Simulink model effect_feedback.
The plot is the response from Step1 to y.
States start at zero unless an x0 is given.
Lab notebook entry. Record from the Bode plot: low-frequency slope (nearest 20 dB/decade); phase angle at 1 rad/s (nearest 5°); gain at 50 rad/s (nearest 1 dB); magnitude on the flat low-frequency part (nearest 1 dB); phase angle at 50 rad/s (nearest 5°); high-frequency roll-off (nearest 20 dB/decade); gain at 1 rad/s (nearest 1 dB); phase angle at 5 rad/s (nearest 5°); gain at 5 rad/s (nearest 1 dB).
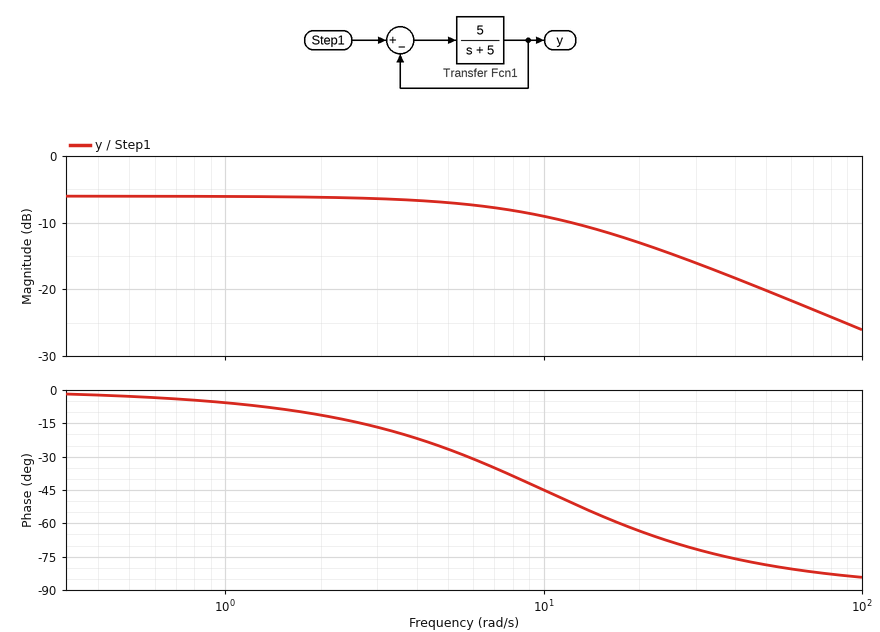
0 dB/decade
-5°
-20 dB
-6 dB
-80°
-20 dB/decade
-6 dB
-25°
-7 dB
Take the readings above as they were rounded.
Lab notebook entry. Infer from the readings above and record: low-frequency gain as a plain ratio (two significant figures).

0.50
